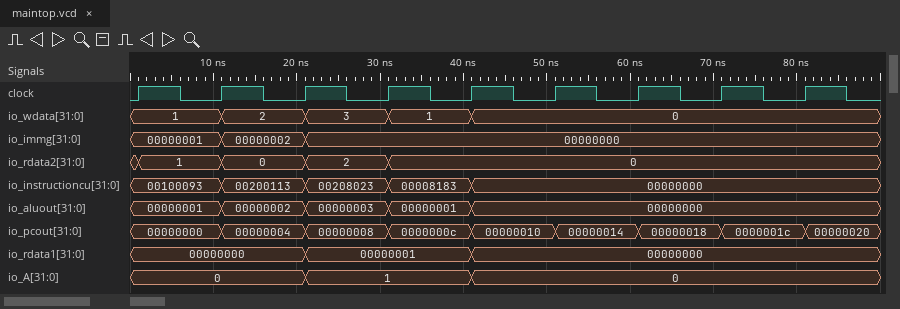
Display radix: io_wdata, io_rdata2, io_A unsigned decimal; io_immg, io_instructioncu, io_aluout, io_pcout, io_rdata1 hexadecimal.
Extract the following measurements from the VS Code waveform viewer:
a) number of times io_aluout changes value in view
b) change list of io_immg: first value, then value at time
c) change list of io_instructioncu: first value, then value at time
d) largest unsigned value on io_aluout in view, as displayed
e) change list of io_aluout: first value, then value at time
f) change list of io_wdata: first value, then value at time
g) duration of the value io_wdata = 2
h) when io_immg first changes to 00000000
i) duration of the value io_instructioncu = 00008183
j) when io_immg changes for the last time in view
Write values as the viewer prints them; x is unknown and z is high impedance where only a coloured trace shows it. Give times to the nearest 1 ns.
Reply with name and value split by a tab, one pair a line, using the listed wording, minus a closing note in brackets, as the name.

number of times io_aluout changes value in view	4
change list of io_immg: first value, then value at time	00000001, 00000002 at 11 ns, 00000000 at 21 ns
change list of io_instructioncu: first value, then value at time	00100093, 00200113 at 11 ns, 00208023 at 21 ns, 00008183 at 31 ns, 00000000 at 41 ns
largest unsigned value on io_aluout in view, as displayed	00000003
change list of io_aluout: first value, then value at time	00000001, 00000002 at 11 ns, 00000003 at 21 ns, 00000001 at 31 ns, 00000000 at 41 ns
change list of io_wdata: first value, then value at time	1, 2 at 11 ns, 3 at 21 ns, 1 at 31 ns, 0 at 41 ns
duration of the value io_wdata = 2	10 ns
when io_immg first changes to 00000000	21 ns
duration of the value io_instructioncu = 00008183	10 ns
when io_immg changes for the last time in view	21 ns
